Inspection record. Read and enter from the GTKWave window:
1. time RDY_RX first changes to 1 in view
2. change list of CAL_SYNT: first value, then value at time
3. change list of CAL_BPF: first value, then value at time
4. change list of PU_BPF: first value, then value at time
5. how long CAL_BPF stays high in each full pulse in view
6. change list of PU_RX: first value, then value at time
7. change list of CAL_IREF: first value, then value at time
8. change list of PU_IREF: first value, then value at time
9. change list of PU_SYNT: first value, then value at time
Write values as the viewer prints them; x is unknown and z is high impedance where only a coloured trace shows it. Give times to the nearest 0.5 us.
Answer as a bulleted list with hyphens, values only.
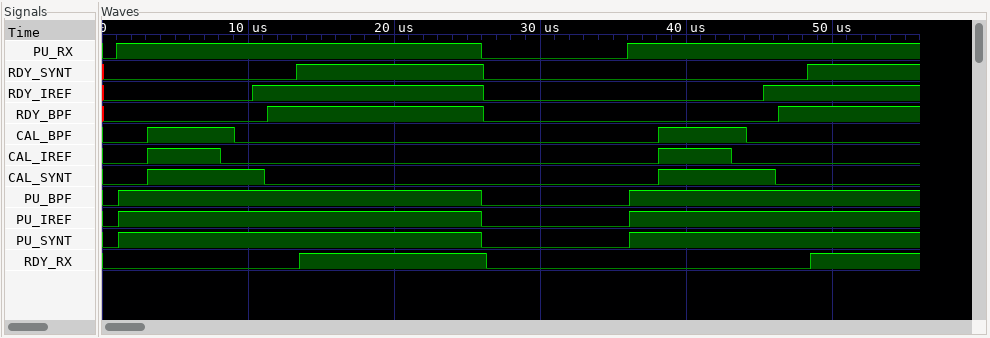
- 13.5 us
- 0, 1 at 3 us, 0 at 11 us, 1 at 38 us, 0 at 46 us
- 0, 1 at 3 us, 0 at 9 us, 1 at 38 us, 0 at 44 us
- 0, 1 at 1 us, 0 at 26 us, 1 at 36 us
- 6 us, 6 us
- 0, 1 at 1 us, 0 at 26 us, 1 at 36 us
- 0, 1 at 3 us, 0 at 8 us, 1 at 38 us, 0 at 43 us
- 0, 1 at 1 us, 0 at 26 us, 1 at 36 us
- 0, 1 at 1 us, 0 at 26 us, 1 at 36 us
